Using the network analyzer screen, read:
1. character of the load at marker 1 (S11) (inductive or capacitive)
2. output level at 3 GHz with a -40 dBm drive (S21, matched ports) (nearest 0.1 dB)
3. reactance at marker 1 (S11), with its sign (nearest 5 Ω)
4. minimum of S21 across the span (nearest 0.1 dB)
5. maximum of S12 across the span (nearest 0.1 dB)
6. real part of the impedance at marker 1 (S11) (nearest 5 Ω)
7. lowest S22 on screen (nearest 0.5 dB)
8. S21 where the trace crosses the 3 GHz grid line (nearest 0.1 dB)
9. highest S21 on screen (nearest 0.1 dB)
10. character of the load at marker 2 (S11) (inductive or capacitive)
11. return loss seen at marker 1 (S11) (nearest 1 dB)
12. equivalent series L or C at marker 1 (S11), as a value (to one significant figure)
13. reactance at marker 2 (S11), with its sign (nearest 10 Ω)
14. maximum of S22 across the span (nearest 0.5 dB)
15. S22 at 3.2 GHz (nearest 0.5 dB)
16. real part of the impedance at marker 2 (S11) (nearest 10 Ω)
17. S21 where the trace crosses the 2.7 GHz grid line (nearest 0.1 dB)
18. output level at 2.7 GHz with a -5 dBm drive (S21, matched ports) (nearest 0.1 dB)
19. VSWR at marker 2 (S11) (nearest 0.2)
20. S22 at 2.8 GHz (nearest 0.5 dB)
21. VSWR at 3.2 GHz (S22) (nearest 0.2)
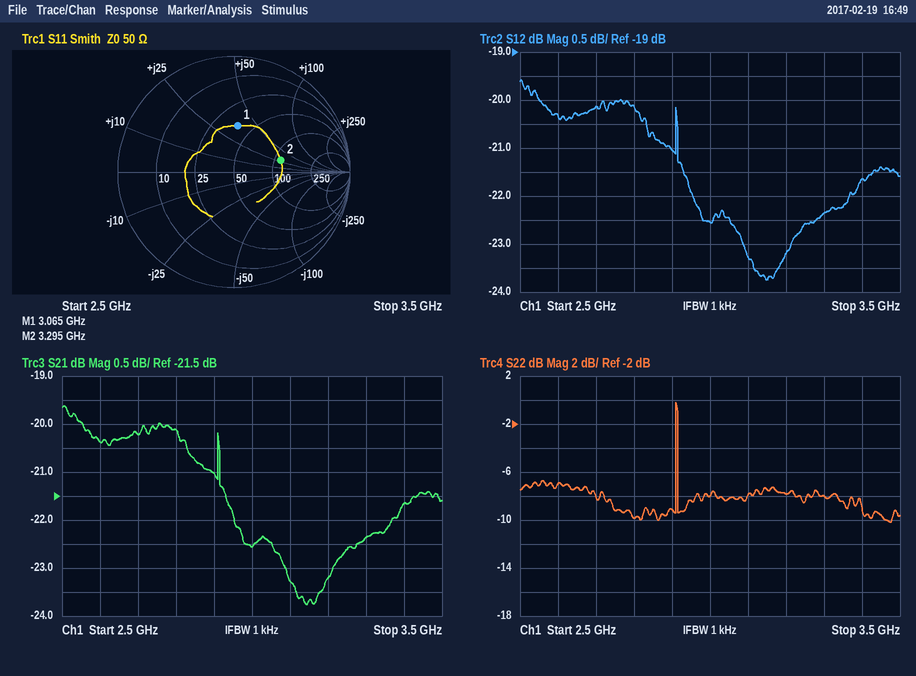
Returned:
inductive
-62.6 dBm
+35 Ω
-23.8 dB
-19.6 dB
40 Ω
-10.0 dB
-22.6 dB
-19.6 dB
inductive
8 dB
2 nH
+30 Ω
0.0 dB
-8.0 dB
110 Ω
-20.2 dB
-25.2 dBm
2.4
-10.0 dB
2.4
